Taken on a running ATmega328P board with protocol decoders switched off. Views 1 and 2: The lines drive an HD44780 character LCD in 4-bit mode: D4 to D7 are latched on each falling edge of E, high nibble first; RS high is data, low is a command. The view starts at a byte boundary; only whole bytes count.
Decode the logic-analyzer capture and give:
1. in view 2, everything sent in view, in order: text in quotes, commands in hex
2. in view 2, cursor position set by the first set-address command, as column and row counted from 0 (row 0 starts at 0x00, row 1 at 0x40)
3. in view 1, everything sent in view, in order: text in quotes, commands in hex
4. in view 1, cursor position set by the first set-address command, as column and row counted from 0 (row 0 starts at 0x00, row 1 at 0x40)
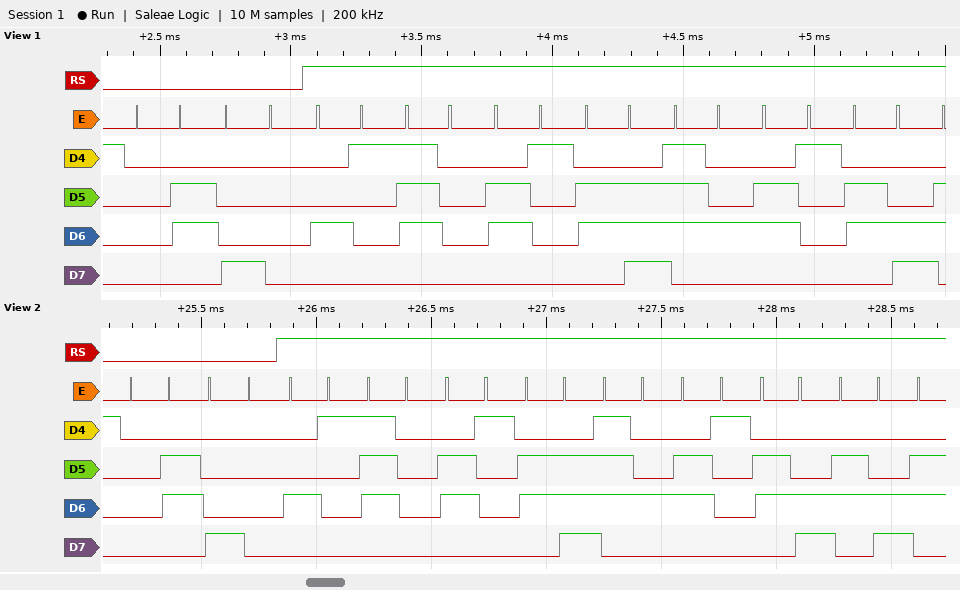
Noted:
0x06 0x80 "Apantall"
column 0, row 0
0x06 0x80 "Apantal"
column 0, row 0
